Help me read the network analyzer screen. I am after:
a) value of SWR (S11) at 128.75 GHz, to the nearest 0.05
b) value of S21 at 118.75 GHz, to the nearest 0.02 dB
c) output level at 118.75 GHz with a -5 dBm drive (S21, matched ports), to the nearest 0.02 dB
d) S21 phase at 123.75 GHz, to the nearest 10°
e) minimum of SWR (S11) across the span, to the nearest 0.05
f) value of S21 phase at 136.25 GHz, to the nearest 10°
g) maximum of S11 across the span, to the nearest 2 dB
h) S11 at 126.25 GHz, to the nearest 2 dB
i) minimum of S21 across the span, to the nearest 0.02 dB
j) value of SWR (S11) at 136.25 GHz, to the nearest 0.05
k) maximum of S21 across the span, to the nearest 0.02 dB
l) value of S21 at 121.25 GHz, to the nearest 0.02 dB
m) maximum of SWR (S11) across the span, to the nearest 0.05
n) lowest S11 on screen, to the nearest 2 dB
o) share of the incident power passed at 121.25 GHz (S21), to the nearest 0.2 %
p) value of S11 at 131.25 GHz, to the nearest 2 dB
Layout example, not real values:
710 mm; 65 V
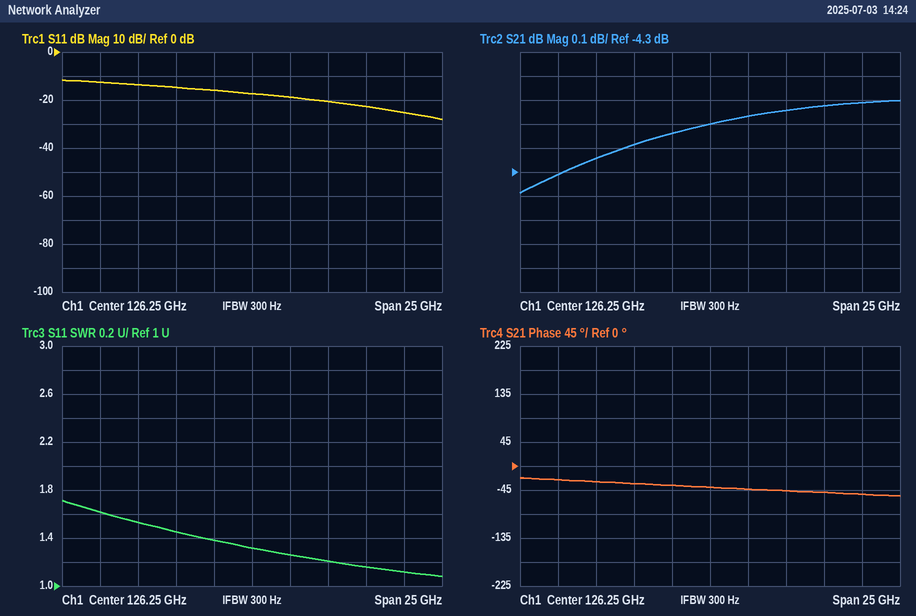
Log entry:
1.25; -4.24 dB; -9.24 dBm; -40°; 1.10; -50°; -12 dB; -18 dB; -4.38 dB; 1.10; -4.00 dB; -4.18 dB; 1.70; -28 dB; 38.2 %; -20 dB
